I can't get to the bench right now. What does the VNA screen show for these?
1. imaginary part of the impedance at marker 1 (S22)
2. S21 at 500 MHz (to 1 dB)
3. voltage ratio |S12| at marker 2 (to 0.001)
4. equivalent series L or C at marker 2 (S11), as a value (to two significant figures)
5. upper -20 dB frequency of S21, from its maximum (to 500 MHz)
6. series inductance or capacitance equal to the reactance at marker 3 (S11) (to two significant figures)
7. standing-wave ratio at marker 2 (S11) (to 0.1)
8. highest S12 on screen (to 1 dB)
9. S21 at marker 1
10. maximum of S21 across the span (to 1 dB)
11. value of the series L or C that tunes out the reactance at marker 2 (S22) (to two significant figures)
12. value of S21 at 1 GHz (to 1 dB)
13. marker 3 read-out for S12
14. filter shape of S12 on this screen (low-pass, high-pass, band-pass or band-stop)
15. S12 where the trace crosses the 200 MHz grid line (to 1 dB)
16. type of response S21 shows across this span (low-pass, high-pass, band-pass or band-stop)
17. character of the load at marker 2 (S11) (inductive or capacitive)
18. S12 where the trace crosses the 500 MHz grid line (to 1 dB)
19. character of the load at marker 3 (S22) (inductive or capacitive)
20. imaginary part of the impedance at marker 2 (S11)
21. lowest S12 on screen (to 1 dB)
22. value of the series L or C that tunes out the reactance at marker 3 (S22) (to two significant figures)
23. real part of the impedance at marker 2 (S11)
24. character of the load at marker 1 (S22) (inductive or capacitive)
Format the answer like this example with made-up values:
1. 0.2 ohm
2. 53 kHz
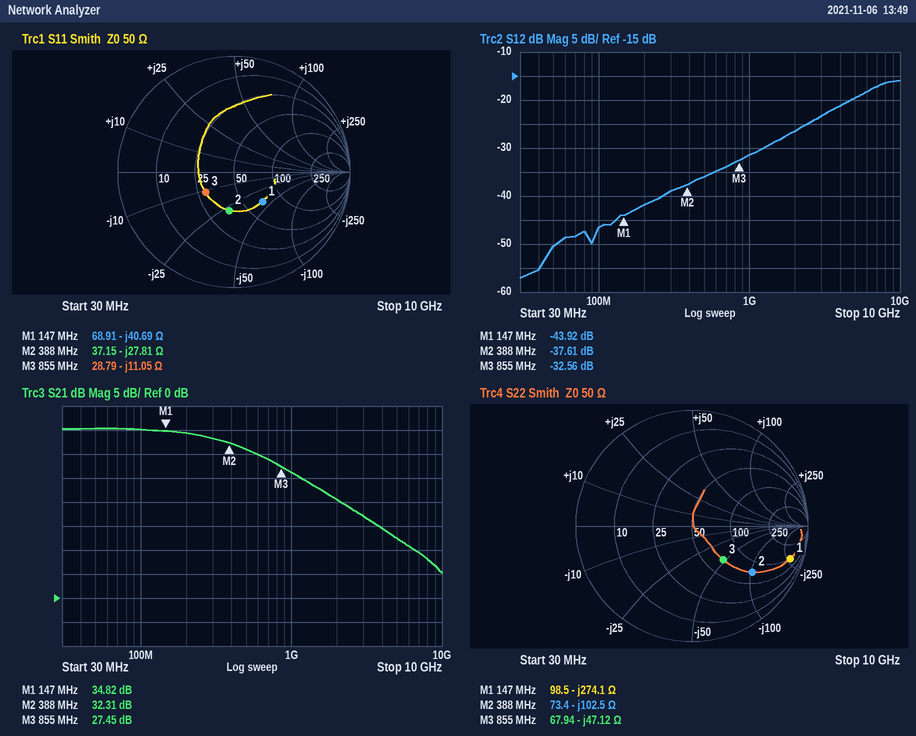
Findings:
1. -274.1 Ω
2. 31 dB
3. 0.013
4. 15 pF
5. 3.5 GHz
6. 17 pF
7. 2.0
8. -16 dB
9. 34.82 dB
10. 35 dB
11. 42 nH
12. 26 dB
13. -32.56 dB
14. high-pass
15. -42 dB
16. low-pass
17. capacitive
18. -36 dB
19. capacitive
20. -27.81 Ω
21. -57 dB
22. 8.8 nH
23. 37.15 Ω
24. capacitive
